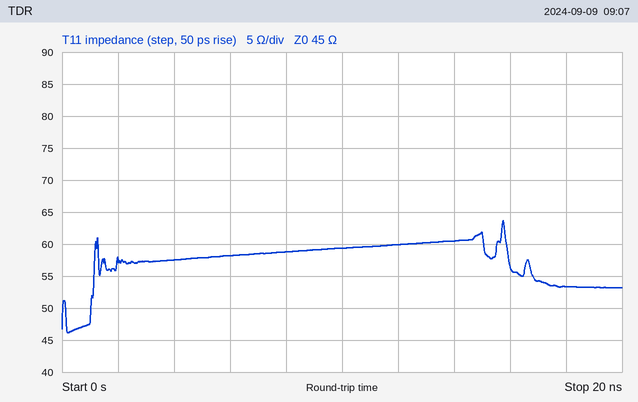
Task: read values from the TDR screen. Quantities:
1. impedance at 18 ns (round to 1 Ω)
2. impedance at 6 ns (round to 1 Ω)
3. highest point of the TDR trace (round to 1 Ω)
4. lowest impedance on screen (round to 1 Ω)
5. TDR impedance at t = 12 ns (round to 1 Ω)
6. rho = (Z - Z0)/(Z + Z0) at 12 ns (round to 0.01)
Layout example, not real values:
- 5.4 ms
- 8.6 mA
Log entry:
- 53 Ω
- 58 Ω
- 64 Ω
- 46 Ω
- 60 Ω
- +0.14
